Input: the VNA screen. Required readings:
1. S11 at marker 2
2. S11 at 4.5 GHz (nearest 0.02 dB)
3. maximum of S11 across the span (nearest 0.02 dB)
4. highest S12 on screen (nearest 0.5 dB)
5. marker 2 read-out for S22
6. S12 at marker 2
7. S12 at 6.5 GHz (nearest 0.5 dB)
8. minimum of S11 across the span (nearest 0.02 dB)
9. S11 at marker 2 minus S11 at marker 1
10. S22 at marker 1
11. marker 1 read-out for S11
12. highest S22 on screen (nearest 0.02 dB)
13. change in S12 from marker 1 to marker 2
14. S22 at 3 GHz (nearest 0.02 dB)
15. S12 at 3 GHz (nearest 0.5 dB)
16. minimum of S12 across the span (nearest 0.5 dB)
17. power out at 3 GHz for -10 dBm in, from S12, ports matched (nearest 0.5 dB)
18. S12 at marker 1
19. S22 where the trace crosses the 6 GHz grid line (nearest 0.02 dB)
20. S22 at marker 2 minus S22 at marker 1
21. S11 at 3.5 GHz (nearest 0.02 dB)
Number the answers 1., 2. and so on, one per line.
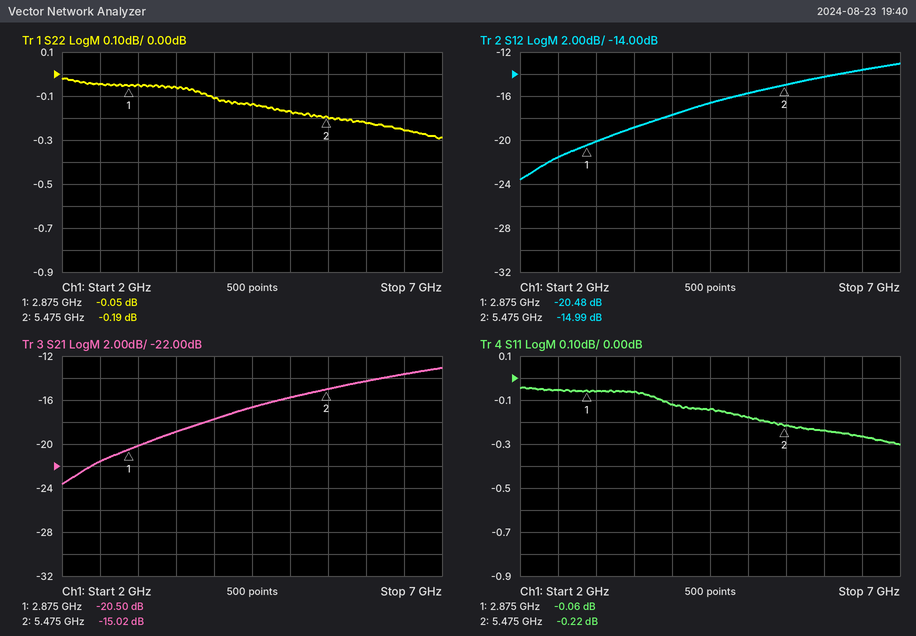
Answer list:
1. -0.22 dB
2. -0.14 dB
3. -0.04 dB
4. -13.0 dB
5. -0.19 dB
6. -14.99 dB
7. -13.5 dB
8. -0.30 dB
9. -0.16 dB
10. -0.05 dB
11. -0.06 dB
12. -0.02 dB
13. 5.49 dB
14. -0.04 dB
15. -20.0 dB
16. -23.5 dB
17. -30.0 dBm
18. -20.48 dB
19. -0.22 dB
20. -0.14 dB
21. -0.06 dB
